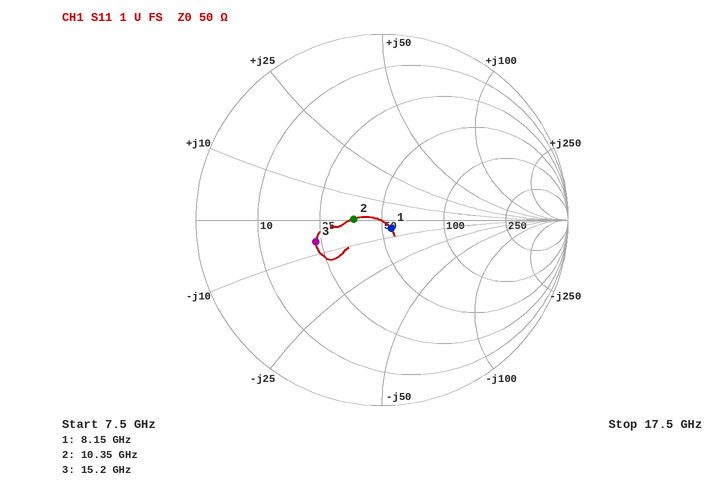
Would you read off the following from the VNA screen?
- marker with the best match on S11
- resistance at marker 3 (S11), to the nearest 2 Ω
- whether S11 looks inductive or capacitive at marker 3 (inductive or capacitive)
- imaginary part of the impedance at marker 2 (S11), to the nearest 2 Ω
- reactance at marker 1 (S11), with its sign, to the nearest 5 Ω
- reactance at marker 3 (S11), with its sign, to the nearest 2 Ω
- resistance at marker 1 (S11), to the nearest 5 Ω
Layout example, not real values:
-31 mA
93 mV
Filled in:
marker 1
24 Ω
capacitive
0 Ω
-5 Ω
-6 Ω
55 Ω
